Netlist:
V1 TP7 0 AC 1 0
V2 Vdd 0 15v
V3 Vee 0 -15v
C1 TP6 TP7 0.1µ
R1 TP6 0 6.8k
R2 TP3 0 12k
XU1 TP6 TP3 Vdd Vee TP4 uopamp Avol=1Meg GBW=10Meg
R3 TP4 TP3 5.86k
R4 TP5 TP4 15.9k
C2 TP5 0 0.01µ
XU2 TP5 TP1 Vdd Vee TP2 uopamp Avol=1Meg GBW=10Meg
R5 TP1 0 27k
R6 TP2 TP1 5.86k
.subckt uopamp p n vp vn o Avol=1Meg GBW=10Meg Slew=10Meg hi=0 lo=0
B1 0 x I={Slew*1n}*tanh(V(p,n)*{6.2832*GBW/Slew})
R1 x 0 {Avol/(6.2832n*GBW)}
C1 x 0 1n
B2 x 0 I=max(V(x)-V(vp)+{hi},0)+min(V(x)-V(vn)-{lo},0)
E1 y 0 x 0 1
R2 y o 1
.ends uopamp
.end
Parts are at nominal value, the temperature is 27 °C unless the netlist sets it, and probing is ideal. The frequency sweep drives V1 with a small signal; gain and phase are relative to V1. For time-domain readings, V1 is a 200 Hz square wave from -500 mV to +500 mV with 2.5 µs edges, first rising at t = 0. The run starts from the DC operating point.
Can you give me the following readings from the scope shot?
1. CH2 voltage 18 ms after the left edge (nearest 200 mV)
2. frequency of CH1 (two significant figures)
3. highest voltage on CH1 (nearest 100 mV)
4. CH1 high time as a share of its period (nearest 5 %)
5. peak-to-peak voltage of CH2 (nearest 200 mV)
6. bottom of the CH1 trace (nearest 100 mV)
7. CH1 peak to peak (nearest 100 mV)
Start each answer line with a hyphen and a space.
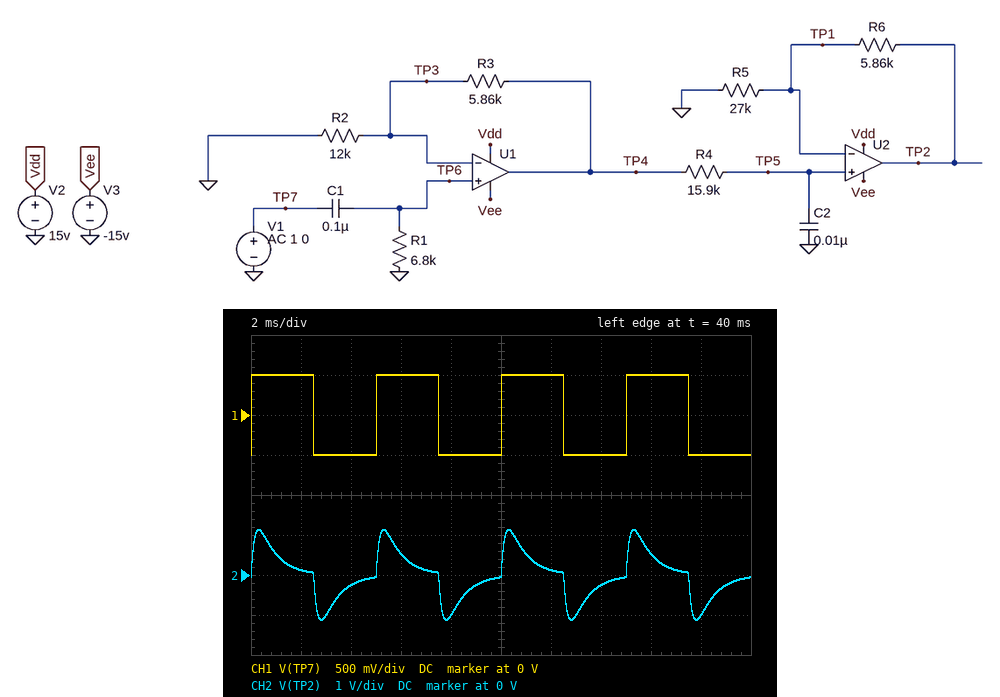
- -1.0 V
- 200 Hz
- 500 mV
- 50 %
- 2.2 V
- -500 mV
- 1.0 V
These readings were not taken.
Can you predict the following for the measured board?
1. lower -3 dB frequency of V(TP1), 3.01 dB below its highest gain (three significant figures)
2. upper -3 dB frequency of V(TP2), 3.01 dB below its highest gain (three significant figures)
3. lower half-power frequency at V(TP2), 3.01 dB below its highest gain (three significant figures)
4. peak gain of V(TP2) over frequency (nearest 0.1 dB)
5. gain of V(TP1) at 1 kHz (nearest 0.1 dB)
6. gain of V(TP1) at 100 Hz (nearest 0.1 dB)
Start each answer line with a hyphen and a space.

- 167 Hz
- 1.40 kHz
- 167 Hz
- 3.3 dB
- 0.2 dB
- -4.7 dB
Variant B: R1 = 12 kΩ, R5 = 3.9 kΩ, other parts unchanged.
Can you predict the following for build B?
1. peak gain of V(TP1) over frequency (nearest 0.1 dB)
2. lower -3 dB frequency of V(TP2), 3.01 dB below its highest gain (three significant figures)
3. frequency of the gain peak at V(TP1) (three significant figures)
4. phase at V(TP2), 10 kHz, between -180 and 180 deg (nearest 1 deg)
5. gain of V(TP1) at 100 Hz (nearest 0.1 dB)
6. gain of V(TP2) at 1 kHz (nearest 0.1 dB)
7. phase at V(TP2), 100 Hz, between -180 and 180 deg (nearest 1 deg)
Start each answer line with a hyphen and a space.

- 2.4 dB
- 107 Hz
- 364 Hz
- -84 deg
- -1.0 dB
- 8.3 dB
- 47 deg
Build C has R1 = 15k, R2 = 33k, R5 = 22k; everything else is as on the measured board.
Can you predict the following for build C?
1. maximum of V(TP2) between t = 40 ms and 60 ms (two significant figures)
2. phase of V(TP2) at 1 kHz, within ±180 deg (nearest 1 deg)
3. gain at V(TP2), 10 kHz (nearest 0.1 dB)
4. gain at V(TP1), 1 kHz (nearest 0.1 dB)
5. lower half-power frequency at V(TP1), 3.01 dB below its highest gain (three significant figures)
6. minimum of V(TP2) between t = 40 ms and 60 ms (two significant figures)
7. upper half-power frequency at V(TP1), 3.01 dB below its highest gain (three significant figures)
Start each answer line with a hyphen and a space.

- 940 mV
- -39 deg
- -16.6 dB
- -1.6 dB
- 88.8 Hz
- -940 mV
- 1.20 kHz
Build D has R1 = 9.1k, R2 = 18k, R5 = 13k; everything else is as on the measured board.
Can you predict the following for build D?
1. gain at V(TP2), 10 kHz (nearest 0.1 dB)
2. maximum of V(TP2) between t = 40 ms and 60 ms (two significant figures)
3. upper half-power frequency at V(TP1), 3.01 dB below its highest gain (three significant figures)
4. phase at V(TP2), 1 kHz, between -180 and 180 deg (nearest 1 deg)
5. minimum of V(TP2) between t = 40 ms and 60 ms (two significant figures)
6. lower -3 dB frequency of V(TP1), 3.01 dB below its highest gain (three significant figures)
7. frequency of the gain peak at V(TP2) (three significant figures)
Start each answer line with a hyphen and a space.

- -14.4 dB
- 1.2 V
- 1.31 kHz
- -35 deg
- -1.2 V
- 134 Hz
- 418 Hz
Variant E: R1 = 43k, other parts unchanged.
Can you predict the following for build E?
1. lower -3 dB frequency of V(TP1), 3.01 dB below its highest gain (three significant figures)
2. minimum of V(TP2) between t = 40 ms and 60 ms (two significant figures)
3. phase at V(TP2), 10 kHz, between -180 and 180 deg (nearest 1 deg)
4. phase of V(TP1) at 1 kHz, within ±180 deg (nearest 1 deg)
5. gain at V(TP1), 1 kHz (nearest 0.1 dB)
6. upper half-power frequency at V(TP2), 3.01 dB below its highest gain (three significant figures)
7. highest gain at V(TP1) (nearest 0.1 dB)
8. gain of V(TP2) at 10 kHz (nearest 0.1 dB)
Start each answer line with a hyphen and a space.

- 34.5 Hz
- -1.0 V
- -84 deg
- -43 deg
- 0.4 dB
- 1.07 kHz
- 3.1 dB
- -14.9 dB
